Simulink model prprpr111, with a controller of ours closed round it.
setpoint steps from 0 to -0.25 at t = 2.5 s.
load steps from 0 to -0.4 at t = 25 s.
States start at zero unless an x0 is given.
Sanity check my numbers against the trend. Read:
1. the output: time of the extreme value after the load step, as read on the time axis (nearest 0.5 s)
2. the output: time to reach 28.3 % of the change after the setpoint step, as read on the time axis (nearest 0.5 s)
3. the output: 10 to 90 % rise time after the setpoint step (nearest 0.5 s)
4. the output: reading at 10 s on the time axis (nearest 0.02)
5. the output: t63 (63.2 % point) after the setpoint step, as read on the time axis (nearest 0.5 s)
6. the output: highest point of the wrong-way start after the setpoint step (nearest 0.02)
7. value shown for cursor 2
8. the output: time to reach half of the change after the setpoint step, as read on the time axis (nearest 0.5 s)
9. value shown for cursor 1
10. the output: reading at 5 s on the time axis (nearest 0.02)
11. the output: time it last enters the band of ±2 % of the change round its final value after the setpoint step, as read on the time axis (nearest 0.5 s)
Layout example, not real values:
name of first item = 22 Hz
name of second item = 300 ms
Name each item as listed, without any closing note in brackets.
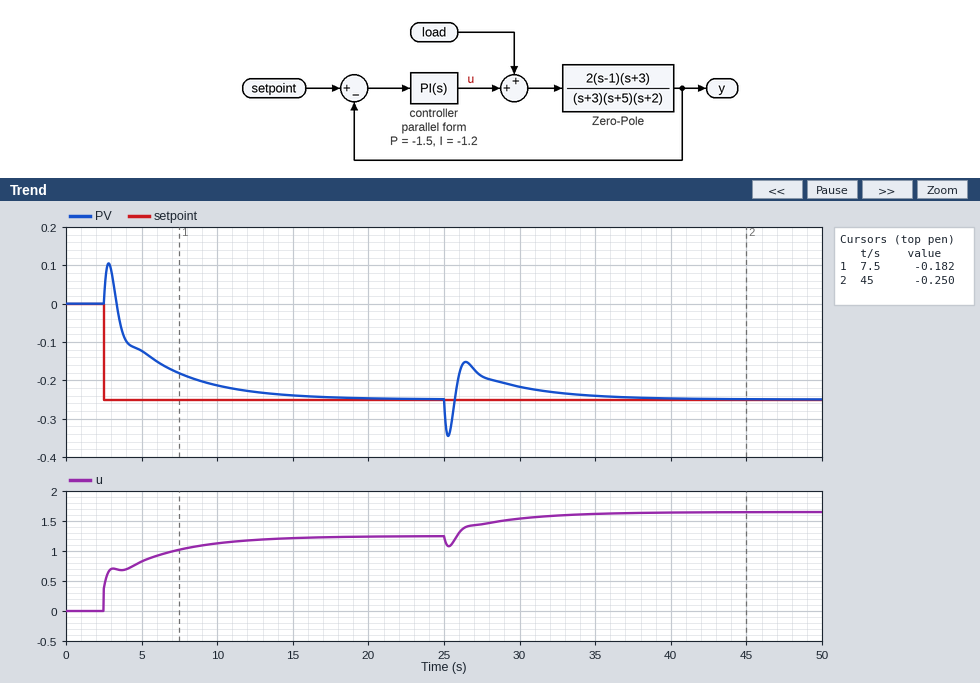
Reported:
the output: time of the extreme value after the load step, as read on the time axis = 26.5 s
the output: time to reach 28.3 % of the change after the setpoint step, as read on the time axis = 3.5 s
the output: 10 to 90 % rise time after the setpoint step = 8.0 s
the output: reading at 10 s on the time axis = -0.22
the output: t63 (63.2 % point) after the setpoint step, as read on the time axis = 6.5 s
the output: highest point of the wrong-way start after the setpoint step = 0.10
value shown for cursor 2 = -0.250
the output: time to reach half of the change after the setpoint step, as read on the time axis = 5.0 s
value shown for cursor 1 = -0.182
the output: reading at 5 s on the time axis = -0.12
the output: time it last enters the band of ±2 % of the change round its final value after the setpoint step, as read on the time axis = 18.0 s
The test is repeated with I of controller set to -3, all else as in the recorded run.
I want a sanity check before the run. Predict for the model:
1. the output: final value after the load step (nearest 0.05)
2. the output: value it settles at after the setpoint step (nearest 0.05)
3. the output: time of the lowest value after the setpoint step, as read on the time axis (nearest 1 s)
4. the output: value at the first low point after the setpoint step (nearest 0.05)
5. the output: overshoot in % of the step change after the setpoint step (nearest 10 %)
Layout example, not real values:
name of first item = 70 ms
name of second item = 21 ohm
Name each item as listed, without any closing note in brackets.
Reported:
the output: final value after the load step = -0.25
the output: value it settles at after the setpoint step = -0.25
the output: time of the lowest value after the setpoint step, as read on the time axis = 5 s
the output: value at the first low point after the setpoint step = -0.30
the output: overshoot in % of the step change after the setpoint step = 20 %
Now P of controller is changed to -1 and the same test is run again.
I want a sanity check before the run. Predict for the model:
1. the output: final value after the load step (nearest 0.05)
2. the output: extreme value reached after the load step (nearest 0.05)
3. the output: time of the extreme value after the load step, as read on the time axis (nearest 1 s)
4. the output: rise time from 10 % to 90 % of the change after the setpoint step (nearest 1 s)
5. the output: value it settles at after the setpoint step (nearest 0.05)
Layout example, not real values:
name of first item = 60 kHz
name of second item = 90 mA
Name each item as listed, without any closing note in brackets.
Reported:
the output: final value after the load step = -0.25
the output: extreme value reached after the load step = -0.15
the output: time of the extreme value after the load step, as read on the time axis = 27 s
the output: rise time from 10 % to 90 % of the change after the setpoint step = 7 s
the output: value it settles at after the setpoint step = -0.25
